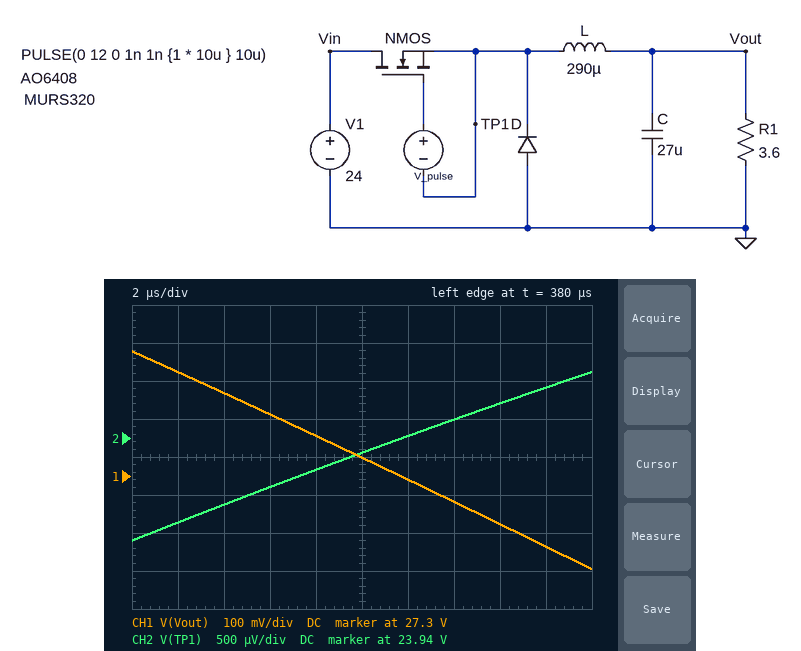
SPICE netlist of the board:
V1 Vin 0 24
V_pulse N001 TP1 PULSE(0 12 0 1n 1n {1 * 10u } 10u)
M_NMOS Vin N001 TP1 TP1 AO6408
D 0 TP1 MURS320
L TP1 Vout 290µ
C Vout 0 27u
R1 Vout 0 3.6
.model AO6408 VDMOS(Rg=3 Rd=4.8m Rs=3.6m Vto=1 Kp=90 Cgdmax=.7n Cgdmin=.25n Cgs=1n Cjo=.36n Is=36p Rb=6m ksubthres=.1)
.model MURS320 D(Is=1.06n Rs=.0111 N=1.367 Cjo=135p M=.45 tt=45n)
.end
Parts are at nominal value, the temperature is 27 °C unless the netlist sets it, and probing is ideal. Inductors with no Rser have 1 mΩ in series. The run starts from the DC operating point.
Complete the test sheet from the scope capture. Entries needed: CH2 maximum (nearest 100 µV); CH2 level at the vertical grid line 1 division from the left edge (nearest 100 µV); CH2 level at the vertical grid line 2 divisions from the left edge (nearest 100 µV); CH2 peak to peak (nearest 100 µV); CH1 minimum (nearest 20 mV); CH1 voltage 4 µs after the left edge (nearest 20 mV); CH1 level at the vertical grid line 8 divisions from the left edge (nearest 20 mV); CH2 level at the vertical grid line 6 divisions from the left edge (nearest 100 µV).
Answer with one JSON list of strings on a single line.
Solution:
["23.9369 V", "23.9349 V", "23.9351 V", "2.2 mV", "27.06 V", "27.52 V", "27.18 V", "23.9360 V"]
